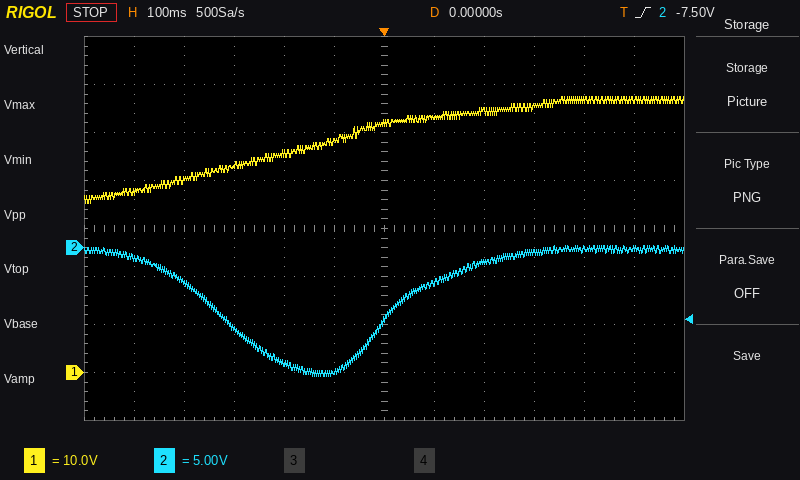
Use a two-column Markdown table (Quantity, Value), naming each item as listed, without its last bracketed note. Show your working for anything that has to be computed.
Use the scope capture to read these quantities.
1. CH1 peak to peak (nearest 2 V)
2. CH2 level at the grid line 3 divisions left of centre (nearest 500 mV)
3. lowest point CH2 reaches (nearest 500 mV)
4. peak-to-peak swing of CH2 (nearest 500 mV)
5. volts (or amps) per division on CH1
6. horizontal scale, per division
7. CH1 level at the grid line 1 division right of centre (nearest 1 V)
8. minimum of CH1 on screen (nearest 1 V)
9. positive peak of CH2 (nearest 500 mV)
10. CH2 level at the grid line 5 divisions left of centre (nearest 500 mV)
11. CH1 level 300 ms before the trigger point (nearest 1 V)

| Quantity | Value |
|---|---|
| CH1 peak to peak | 22 V |
| CH2 level at the grid line 3 divisions left of centre | -8.5 V |
| lowest point CH2 reaches | -13.5 V |
| peak-to-peak swing of CH2 | 0.0 V − (-13.5 V) = 13.5 V |
| volts (or amps) per division on CH1 | 10 V |
| horizontal scale, per division | 100 ms |
| CH1 level at the grid line 1 division right of centre | 53 V |
| minimum of CH1 on screen | 35 V |
| positive peak of CH2 | 0.0 V |
| CH2 level at the grid line 5 divisions left of centre | -1.0 V |
| CH1 level 300 ms before the trigger point | 43 V |
